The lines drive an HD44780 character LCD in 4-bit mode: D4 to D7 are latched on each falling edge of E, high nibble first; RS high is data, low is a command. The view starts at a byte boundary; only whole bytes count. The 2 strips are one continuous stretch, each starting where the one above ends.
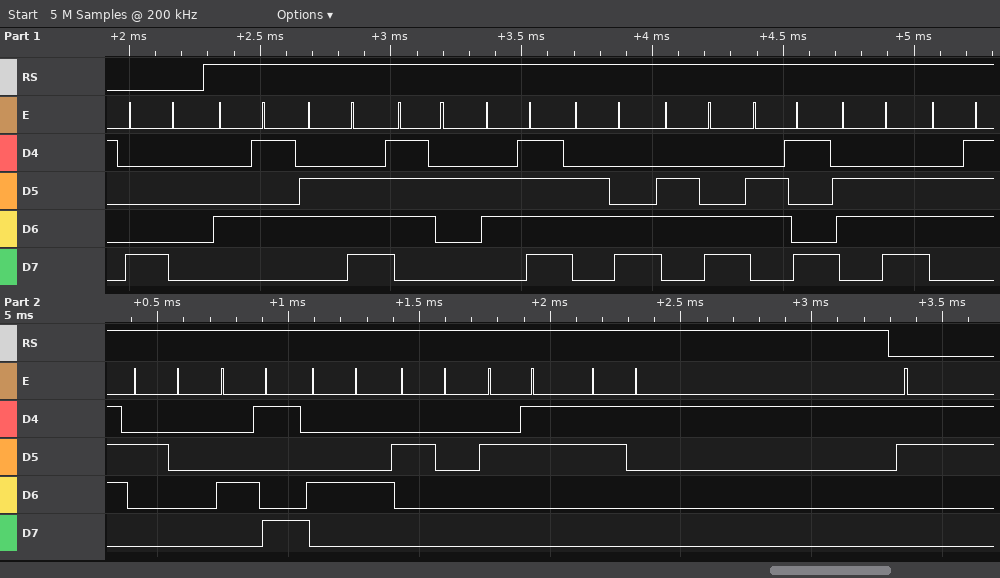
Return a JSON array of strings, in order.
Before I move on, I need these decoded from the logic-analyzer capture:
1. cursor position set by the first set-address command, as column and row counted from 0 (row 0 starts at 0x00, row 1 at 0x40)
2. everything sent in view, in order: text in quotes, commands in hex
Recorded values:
["column 0, row 0", "0x80 \"Enrolling ID #1\""]
